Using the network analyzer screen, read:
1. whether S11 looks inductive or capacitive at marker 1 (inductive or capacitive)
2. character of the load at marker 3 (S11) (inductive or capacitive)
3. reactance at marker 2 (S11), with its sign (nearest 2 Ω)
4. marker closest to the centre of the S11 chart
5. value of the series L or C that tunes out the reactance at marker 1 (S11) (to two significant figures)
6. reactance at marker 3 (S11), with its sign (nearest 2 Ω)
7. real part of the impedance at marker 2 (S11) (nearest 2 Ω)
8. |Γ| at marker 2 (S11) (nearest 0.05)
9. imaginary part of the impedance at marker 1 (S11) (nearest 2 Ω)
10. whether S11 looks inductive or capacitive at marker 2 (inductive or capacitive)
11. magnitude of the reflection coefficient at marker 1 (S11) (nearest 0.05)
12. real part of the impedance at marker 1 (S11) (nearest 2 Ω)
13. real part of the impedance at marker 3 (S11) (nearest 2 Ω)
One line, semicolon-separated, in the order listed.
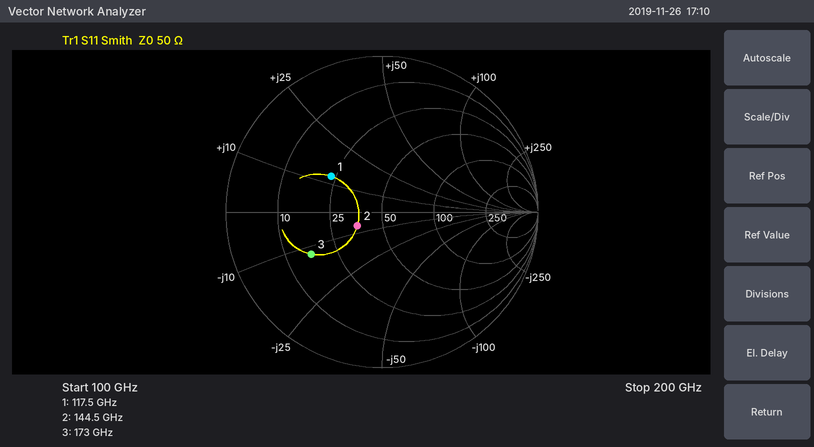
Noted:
inductive; capacitive; -6 Ω; marker 2; 110 fF; -12 Ω; 36 Ω; 0.20; +12 Ω; capacitive; 0.40; 24 Ω; 16 Ω
